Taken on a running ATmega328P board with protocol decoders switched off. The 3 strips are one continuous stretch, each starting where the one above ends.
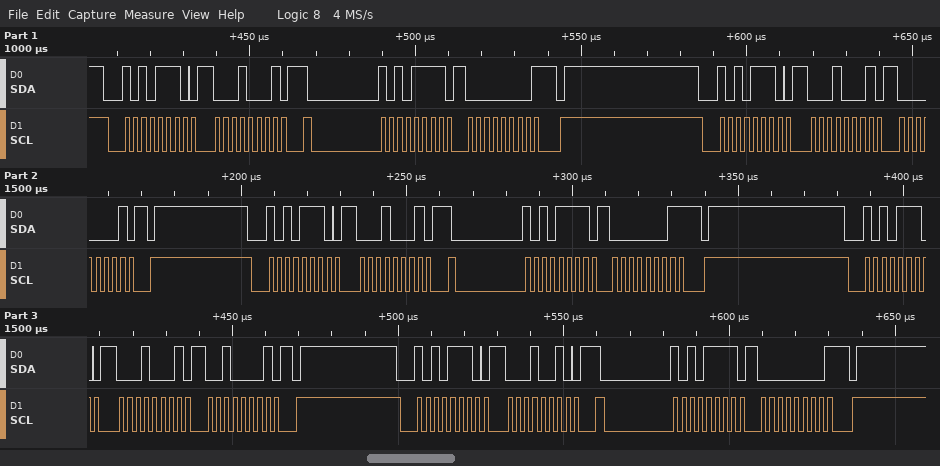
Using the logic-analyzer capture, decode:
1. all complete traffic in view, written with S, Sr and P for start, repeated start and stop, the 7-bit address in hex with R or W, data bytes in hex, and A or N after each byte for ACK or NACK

S 57W A 11 A Sr 57R A 00 N P S 57W A 11 A 01 A P S 57W A 11 A Sr 57R A 01 N P S 57W A 11 A 21 A P S 57W A 12 A Sr 57R A 00 N P
